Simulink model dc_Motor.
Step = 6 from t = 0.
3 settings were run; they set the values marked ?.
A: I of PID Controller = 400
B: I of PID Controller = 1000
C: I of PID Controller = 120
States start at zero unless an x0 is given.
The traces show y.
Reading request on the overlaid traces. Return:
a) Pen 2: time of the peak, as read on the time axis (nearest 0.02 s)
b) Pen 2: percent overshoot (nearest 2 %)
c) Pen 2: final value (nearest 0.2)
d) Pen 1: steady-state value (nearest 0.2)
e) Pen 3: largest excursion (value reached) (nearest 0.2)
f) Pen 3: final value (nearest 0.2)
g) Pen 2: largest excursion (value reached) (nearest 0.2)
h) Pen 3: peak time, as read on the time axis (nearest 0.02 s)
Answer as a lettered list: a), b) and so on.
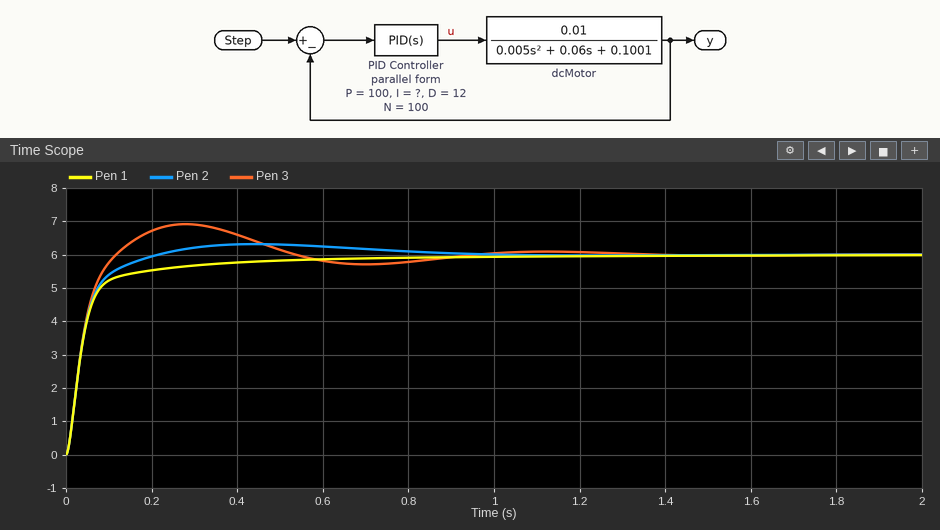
a) 0.44 s
b) 6 %
c) 6.0
d) 6.0
e) 7.0
f) 6.0
g) 6.4
h) 0.28 s
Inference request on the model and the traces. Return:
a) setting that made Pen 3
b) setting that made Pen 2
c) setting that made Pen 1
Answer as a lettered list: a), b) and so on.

a) B
b) A
c) C
